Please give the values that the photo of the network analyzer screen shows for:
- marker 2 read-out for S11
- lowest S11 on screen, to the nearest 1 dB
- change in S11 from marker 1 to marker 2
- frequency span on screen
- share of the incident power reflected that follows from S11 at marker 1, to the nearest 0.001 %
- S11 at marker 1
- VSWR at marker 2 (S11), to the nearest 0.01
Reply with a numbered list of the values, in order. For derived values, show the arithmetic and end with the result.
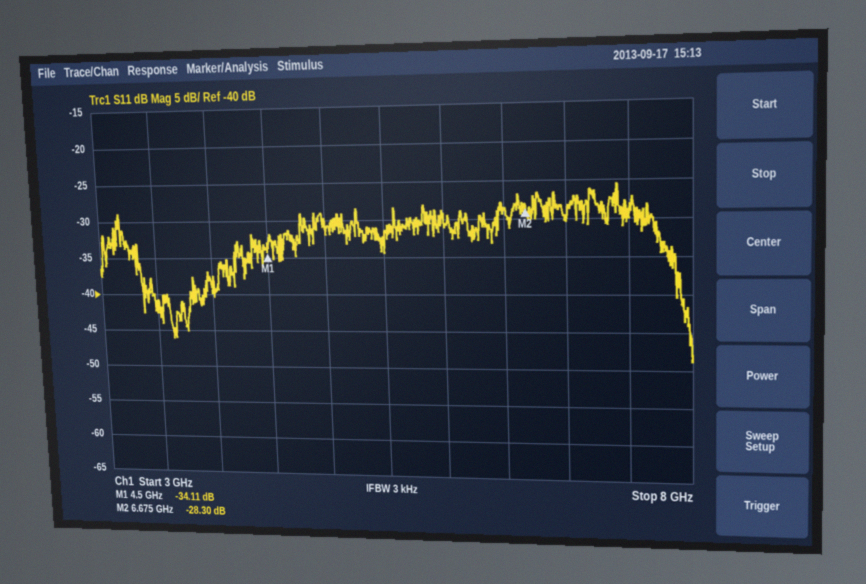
1. -28.30 dB
2. -49 dB
3. -28.3 − (-34.11) = 5.81 dB
4. 5 GHz
5. 10^(-34.11/10) ≈ 0.039 %
6. -34.11 dB
7. (1 + 0.0385)/(1 − 0.0385) ≈ 1.08
